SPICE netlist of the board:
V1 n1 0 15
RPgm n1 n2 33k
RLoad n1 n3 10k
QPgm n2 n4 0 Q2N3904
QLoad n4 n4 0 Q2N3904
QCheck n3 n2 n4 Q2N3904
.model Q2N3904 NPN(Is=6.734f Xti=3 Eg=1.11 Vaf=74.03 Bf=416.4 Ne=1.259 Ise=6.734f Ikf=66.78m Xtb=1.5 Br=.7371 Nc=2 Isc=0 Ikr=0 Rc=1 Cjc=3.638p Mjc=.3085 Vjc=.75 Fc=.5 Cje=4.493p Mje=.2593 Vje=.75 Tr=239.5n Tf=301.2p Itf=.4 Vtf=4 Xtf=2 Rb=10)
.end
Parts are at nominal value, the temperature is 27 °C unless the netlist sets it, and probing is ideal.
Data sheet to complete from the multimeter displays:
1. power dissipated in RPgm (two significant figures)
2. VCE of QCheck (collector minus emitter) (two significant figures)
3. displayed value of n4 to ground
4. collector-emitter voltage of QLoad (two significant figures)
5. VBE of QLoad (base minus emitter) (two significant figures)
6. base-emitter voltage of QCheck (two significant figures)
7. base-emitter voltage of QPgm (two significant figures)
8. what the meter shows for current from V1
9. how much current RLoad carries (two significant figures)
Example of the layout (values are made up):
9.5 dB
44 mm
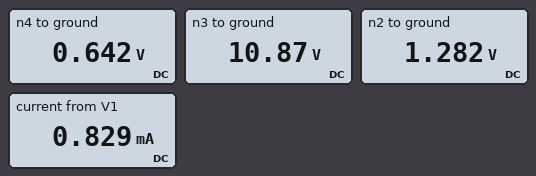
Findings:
5.7 mW
10 V
0.642 V
640 mV
640 mV
640 mV
640 mV
0.829 mA
410 µA
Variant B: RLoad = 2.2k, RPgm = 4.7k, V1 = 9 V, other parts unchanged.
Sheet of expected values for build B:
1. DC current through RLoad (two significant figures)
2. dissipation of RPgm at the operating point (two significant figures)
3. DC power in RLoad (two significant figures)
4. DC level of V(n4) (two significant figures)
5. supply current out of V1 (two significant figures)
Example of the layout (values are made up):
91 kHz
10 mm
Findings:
1.6 mA
12 mW
5.7 mW
680 mV
3.2 mA
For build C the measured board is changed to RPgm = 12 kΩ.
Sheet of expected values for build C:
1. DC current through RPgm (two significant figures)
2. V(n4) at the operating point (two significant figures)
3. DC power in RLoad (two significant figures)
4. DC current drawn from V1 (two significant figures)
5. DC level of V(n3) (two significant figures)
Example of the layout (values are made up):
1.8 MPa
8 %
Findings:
1.1 mA
670 mV
13 mW
2.3 mA
3.7 V
